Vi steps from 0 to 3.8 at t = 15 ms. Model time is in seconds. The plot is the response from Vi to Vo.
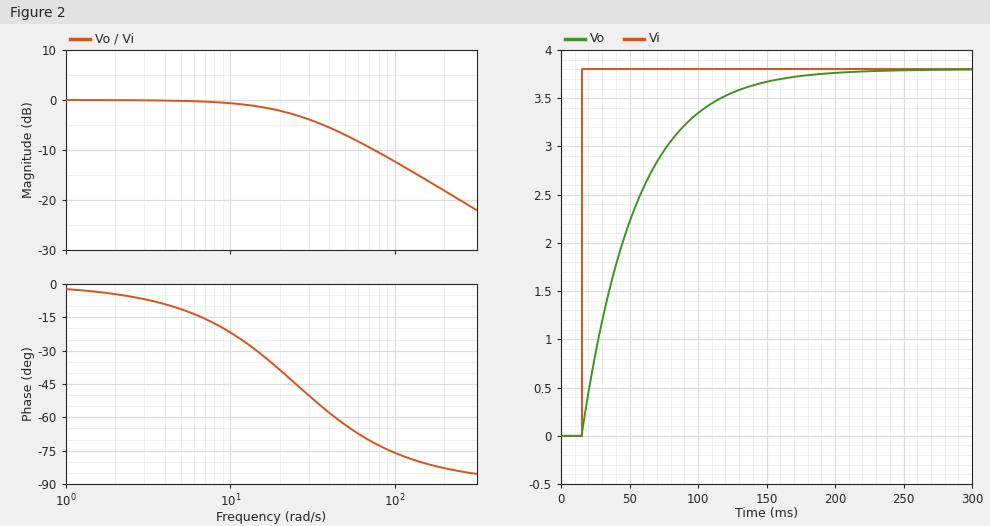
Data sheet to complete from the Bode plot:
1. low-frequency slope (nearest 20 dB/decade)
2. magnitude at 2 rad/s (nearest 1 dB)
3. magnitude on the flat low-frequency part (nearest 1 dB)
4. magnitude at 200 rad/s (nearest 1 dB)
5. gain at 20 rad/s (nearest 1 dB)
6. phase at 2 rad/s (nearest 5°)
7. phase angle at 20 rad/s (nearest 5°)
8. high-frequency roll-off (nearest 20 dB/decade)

0 dB/decade
0 dB
0 dB
-18 dB
-2 dB
-5°
-40°
-20 dB/decade
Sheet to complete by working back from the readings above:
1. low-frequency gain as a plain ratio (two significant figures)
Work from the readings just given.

1.0
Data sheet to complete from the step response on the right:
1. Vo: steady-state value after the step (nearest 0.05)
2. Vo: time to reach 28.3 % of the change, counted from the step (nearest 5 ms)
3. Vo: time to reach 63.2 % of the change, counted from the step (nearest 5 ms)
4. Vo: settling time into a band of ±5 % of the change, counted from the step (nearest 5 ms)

3.80
15 ms
40 ms
120 ms
